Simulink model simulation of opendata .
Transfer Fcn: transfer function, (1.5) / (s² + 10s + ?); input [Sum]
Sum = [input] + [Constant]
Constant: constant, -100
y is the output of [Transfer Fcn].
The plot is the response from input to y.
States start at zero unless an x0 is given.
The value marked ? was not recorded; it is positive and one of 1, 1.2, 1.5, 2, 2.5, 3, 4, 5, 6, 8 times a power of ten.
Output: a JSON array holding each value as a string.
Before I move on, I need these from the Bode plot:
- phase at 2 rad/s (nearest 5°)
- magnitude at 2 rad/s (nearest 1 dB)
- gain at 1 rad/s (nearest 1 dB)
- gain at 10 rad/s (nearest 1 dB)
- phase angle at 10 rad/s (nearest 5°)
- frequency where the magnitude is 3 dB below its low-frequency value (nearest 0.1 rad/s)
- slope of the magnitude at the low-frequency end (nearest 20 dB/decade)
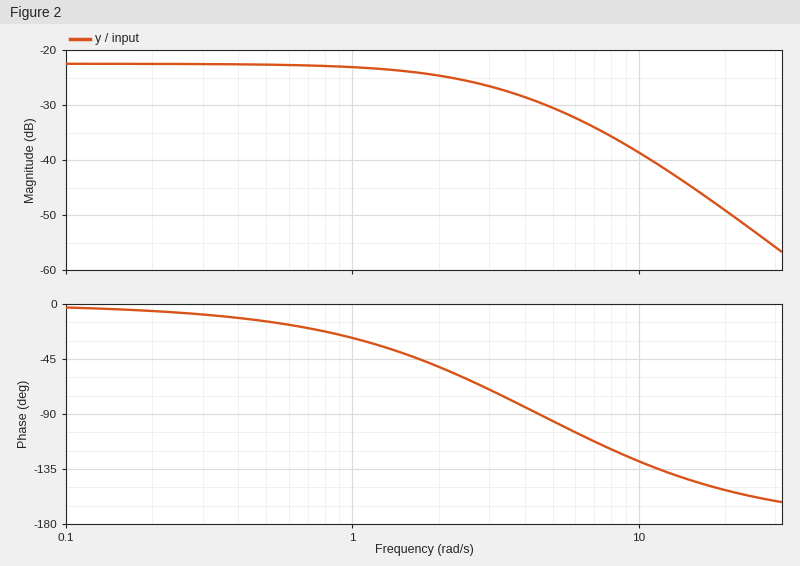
["-50°", "-25 dB", "-23 dB", "-39 dB", "-130°", "2.5 rad/s", "0 dB/decade"]
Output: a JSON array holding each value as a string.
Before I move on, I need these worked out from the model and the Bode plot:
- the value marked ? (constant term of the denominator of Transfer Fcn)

["20"]
